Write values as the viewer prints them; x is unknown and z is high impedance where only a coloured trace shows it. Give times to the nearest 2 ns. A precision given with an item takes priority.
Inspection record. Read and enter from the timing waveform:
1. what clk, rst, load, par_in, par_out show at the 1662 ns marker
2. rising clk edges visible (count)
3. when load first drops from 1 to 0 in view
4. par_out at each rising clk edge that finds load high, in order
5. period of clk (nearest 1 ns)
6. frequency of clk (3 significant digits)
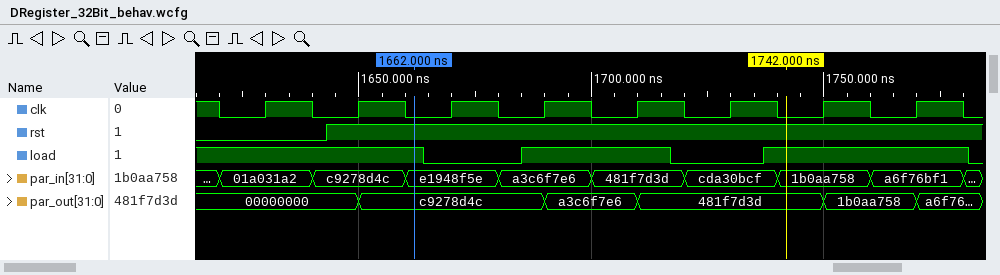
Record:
clk=0, rst=1, load=1, par_in=e1948f5e, par_out=c9278d4c
8
1664 ns
00000000, 00000000, c9278d4c, a3c6f7e6, 481f7d3d, 1b0aa758
20 ns
50.0 MHz
